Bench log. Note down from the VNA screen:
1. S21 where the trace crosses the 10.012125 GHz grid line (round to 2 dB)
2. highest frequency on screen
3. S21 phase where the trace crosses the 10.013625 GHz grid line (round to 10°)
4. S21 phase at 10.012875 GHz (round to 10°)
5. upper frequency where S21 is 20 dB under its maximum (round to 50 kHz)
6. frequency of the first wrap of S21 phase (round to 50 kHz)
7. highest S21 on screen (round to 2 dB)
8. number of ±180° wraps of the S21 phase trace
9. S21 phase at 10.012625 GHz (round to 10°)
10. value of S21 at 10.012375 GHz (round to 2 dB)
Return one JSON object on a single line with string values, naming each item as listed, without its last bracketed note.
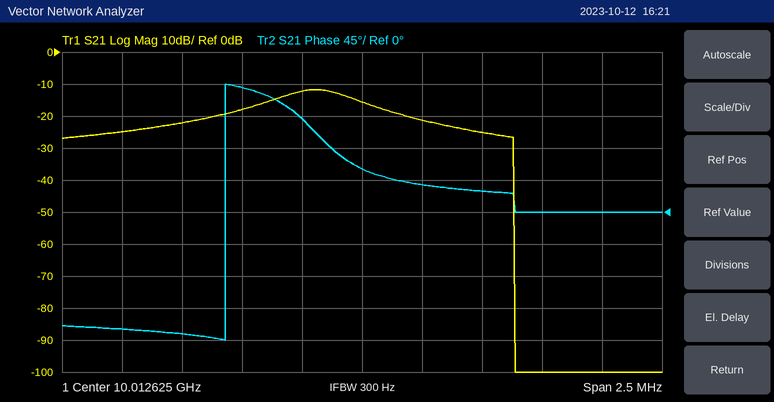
{"S21 where the trace crosses the 10.012125 GHz grid line": "-18 dB", "highest frequency on screen": "10.013875 GHz", "S21 phase where the trace crosses the 10.013625 GHz grid line": "0°", "S21 phase at 10.012875 GHz": "40°", "upper frequency where S21 is 20 dB under its maximum": "10.01325 GHz", "frequency of the first wrap of S21 phase": "10.01205 GHz", "highest S21 on screen": "-12 dB", "number of ±180° wraps of the S21 phase trace": "1", "S21 phase at 10.012625 GHz": "60°", "value of S21 at 10.012375 GHz": "-12 dB"}
